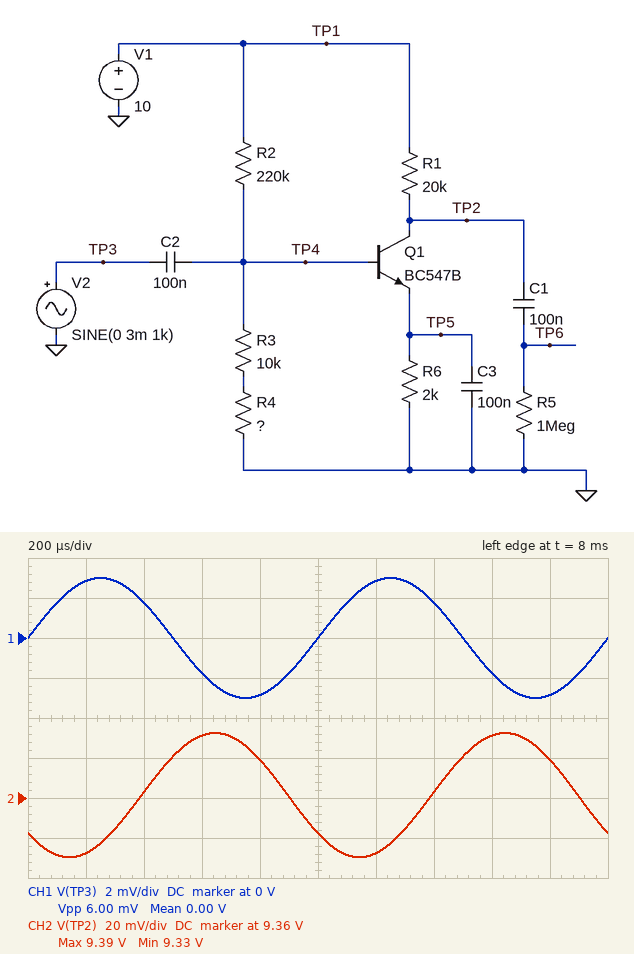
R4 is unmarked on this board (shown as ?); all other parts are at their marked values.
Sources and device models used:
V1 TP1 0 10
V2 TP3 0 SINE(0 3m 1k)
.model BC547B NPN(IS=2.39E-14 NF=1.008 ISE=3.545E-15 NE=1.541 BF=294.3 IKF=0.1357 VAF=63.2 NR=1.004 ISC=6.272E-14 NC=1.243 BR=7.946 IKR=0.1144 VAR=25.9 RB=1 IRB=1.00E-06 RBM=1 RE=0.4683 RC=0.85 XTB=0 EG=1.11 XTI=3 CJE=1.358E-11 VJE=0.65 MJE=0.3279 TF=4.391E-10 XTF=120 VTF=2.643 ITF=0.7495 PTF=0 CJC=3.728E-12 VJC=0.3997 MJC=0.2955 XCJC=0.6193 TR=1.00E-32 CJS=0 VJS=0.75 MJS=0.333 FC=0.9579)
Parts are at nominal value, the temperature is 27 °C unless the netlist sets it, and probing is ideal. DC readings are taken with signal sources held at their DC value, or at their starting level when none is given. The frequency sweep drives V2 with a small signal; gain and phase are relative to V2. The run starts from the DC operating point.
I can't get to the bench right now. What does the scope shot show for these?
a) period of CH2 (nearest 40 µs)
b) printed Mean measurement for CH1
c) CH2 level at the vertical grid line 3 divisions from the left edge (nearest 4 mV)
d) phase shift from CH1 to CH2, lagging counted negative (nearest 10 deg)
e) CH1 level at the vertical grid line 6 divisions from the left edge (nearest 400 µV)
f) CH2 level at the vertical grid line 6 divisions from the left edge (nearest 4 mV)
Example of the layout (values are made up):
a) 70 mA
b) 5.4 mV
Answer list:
a) 1.00 ms
b) 0.00 V
c) 9.392 V
d) -140 deg
e) 2.8 mV
f) 9.332 V
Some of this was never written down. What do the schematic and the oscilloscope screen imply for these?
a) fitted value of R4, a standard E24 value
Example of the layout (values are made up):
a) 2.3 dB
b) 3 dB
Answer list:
a) 4.3 kΩ
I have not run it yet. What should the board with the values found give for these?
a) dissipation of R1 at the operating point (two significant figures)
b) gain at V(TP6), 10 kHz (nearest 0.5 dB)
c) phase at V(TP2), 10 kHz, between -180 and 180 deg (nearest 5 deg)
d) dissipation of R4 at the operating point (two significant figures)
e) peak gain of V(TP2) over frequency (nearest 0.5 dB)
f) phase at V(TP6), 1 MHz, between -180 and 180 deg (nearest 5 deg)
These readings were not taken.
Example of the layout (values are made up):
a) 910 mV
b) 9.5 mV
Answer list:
a) 20 µW
b) 27.0 dB
c) -170 deg
d) 7.8 µW
e) 27.5 dB
f) 170 deg
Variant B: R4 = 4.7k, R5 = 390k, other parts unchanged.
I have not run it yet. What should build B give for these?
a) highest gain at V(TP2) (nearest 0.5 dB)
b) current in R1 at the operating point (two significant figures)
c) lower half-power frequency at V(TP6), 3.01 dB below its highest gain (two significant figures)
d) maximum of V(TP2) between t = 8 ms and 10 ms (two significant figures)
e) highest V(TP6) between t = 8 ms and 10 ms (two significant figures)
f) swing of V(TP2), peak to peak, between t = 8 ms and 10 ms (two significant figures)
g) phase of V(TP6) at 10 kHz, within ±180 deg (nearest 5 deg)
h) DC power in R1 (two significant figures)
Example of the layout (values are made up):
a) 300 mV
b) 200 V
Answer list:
a) 28.5 dB
b) 38 µA
c) 2.9 kHz
d) 9.3 V
e) 32 mV
f) 64 mV
g) -165 deg
h) 28 µW
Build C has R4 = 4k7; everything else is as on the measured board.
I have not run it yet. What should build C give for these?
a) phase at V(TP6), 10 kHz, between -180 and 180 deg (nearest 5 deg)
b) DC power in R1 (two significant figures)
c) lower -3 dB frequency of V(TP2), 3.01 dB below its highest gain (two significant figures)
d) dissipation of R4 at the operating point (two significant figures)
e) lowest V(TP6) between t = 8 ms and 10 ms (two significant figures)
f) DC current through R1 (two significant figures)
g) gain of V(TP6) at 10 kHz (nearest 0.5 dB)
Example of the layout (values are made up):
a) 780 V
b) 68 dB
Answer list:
a) -165 deg
b) 28 µW
c) 2.9 kHz
d) 8.5 µW
e) -33 mV
f) 38 µA
g) 28.5 dB
